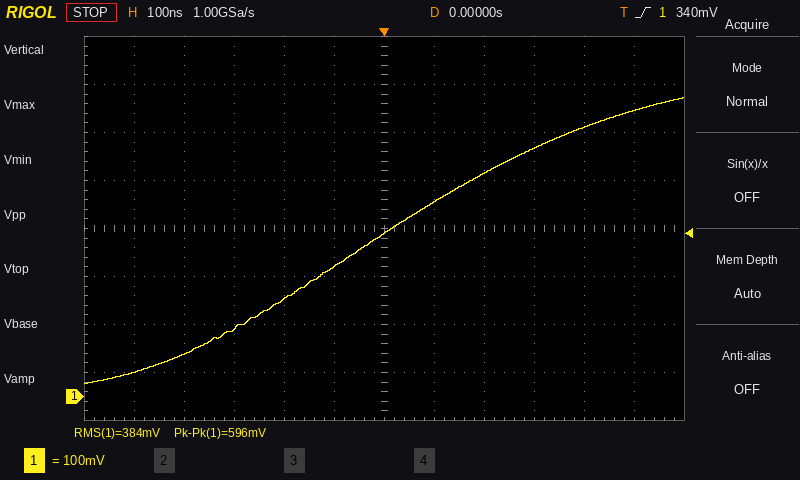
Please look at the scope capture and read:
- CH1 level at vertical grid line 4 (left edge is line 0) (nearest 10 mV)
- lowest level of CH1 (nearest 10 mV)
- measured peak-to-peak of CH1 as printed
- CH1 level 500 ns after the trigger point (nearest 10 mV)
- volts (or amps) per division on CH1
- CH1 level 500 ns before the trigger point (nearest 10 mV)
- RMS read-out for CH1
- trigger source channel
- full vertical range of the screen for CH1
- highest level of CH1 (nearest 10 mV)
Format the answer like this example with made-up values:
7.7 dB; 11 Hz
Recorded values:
200 mV; 30 mV; 596 mV; 600 mV; 100 mV; 50 mV; 384 mV; CH1; 800 mV; 620 mV
